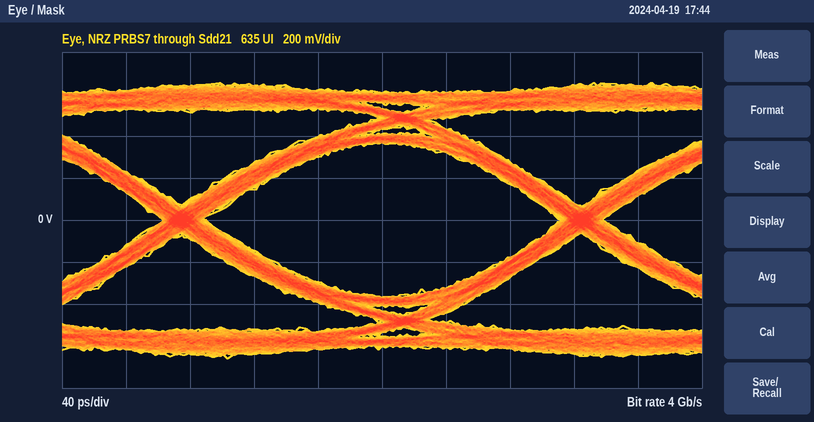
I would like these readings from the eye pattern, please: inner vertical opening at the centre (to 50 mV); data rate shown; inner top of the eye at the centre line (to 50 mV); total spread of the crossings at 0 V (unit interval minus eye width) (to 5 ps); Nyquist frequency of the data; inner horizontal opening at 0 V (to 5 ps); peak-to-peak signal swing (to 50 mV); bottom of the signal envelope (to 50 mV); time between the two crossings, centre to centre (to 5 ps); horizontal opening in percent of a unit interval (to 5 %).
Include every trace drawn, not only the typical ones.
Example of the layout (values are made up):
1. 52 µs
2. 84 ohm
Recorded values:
1. 750 mV
2. 4 Gb/s
3. 350 mV
4. 30 ps
5. 2 GHz
6. 220 ps
7. 1.30 V
8. -650 mV
9. 250 ps
10. 90 %
